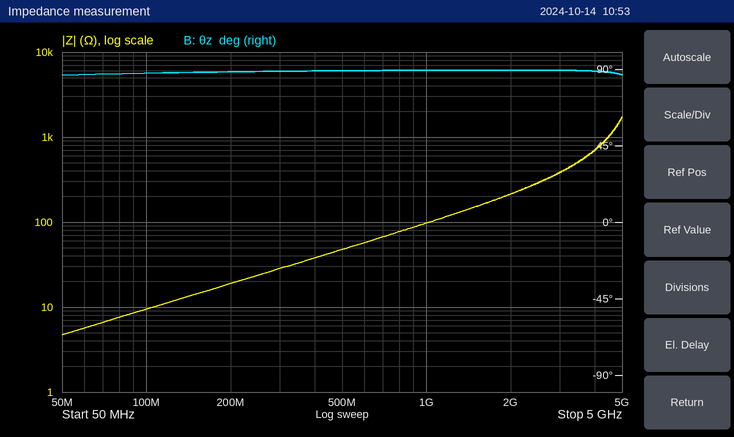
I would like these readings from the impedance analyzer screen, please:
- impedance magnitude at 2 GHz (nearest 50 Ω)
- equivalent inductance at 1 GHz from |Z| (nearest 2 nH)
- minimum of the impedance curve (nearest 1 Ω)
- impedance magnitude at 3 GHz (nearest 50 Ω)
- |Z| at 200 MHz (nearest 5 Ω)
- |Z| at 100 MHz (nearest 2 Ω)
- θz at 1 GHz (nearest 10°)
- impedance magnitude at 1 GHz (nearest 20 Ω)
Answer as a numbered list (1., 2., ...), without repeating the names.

1. 200 Ω
2. 16 nH
3. 5 Ω
4. 400 Ω
5. 20 Ω
6. 10 Ω
7. 90°
8. 100 Ω
